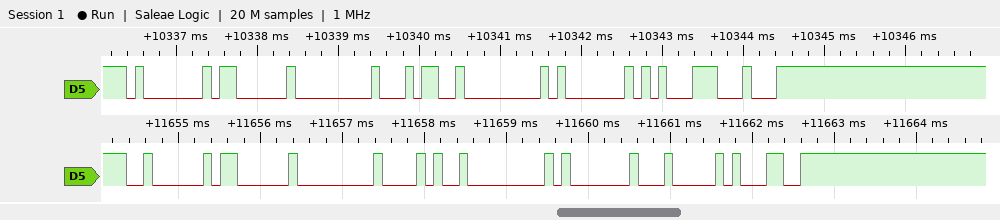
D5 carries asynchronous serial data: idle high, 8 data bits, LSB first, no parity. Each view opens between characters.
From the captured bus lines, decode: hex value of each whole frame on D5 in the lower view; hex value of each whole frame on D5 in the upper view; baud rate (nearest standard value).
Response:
02, 03, 00, 28, 00, 01, 04, 31
01, 03, 00, 34, 00, 01, C5, C4
9600 baud
